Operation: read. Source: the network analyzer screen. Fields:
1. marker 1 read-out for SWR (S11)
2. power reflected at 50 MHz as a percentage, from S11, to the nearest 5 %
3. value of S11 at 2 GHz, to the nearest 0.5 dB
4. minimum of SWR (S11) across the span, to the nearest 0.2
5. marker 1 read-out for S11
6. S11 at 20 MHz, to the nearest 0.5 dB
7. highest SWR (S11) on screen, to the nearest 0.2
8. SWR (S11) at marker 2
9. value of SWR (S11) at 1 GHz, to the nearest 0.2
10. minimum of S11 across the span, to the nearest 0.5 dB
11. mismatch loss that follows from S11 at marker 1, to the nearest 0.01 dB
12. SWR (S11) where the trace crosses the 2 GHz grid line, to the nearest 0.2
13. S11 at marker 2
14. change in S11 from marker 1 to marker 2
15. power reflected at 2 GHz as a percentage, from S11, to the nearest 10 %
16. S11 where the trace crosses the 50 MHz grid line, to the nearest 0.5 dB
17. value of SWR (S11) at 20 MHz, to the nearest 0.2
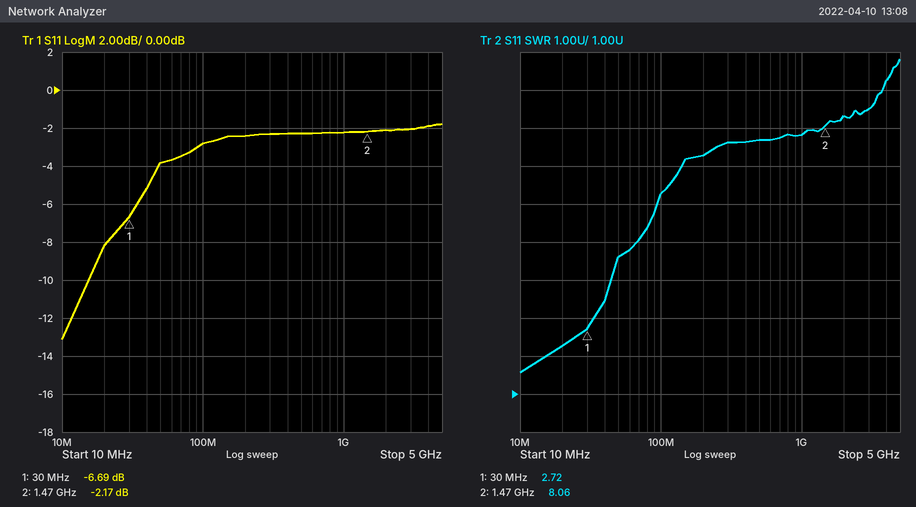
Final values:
2.72
40 %
-2.0 dB
1.6
-6.69 dB
-8.0 dB
9.8
8.06
7.8
-13.0 dB
1.05 dB
8.4
-2.17 dB
4.52 dB
60 %
-4.0 dB
2.2
